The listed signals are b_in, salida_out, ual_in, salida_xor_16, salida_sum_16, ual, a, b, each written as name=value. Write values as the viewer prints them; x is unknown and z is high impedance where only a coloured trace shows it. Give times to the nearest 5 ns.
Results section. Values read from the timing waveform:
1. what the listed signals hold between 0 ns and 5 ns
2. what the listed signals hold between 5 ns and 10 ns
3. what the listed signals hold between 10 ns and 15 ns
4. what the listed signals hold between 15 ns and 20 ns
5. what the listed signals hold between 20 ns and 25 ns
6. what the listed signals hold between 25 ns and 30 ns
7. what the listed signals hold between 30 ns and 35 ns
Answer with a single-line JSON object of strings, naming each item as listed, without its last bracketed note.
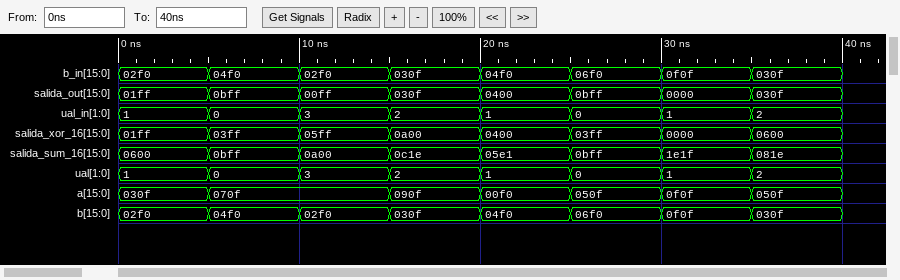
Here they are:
{"what the listed signals hold between 0 ns and 5 ns": "b_in=02f0, salida_out=01ff, ual_in=1, salida_xor_16=01ff, salida_sum_16=0600, ual=1, a=030f, b=02f0", "what the listed signals hold between 5 ns and 10 ns": "b_in=04f0, salida_out=0bff, ual_in=0, salida_xor_16=03ff, salida_sum_16=0bff, ual=0, a=070f, b=04f0", "what the listed signals hold between 10 ns and 15 ns": "b_in=02f0, salida_out=00ff, ual_in=3, salida_xor_16=05ff, salida_sum_16=0a00, ual=3, a=070f, b=02f0", "what the listed signals hold between 15 ns and 20 ns": "b_in=030f, salida_out=030f, ual_in=2, salida_xor_16=0a00, salida_sum_16=0c1e, ual=2, a=090f, b=030f", "what the listed signals hold between 20 ns and 25 ns": "b_in=04f0, salida_out=0400, ual_in=1, salida_xor_16=0400, salida_sum_16=05e1, ual=1, a=00f0, b=04f0", "what the listed signals hold between 25 ns and 30 ns": "b_in=06f0, salida_out=0bff, ual_in=0, salida_xor_16=03ff, salida_sum_16=0bff, ual=0, a=050f, b=06f0", "what the listed signals hold between 30 ns and 35 ns": "b_in=0f0f, salida_out=0000, ual_in=1, salida_xor_16=0000, salida_sum_16=1e1f, ual=1, a=0f0f, b=0f0f"}
